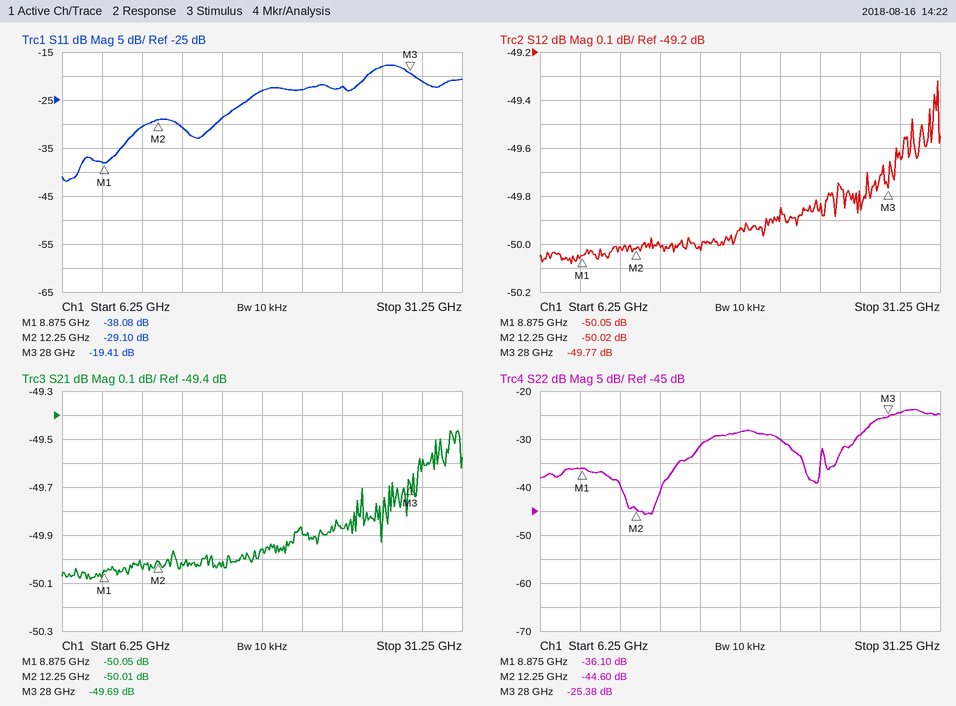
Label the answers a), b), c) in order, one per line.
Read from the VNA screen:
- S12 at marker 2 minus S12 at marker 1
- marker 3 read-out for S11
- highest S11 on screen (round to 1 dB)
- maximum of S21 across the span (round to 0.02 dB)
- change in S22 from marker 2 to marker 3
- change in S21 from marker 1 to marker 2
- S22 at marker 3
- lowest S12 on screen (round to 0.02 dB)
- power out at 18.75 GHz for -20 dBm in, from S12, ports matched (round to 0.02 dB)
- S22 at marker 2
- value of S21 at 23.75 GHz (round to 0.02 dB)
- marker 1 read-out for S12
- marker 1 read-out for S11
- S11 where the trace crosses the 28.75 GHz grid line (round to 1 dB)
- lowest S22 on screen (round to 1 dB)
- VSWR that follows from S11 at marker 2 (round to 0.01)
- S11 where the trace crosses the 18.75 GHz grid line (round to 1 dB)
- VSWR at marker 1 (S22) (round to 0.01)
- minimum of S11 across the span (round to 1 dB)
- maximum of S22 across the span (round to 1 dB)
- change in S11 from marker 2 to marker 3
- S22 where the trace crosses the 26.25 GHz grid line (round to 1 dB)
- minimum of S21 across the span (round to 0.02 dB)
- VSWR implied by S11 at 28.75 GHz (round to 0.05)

a) 0.03 dB
b) -19.41 dB
c) -18 dB
d) -49.46 dB
e) 19.22 dB
f) 0.04 dB
g) -25.38 dB
h) -50.08 dB
i) -69.94 dBm
j) -44.60 dB
k) -49.88 dB
l) -50.05 dB
m) -38.08 dB
n) -21 dB
o) -46 dB
p) 1.07
q) -23 dB
r) 1.03
s) -42 dB
t) -24 dB
u) 9.69 dB
v) -29 dB
w) -50.08 dB
x) 1.20
